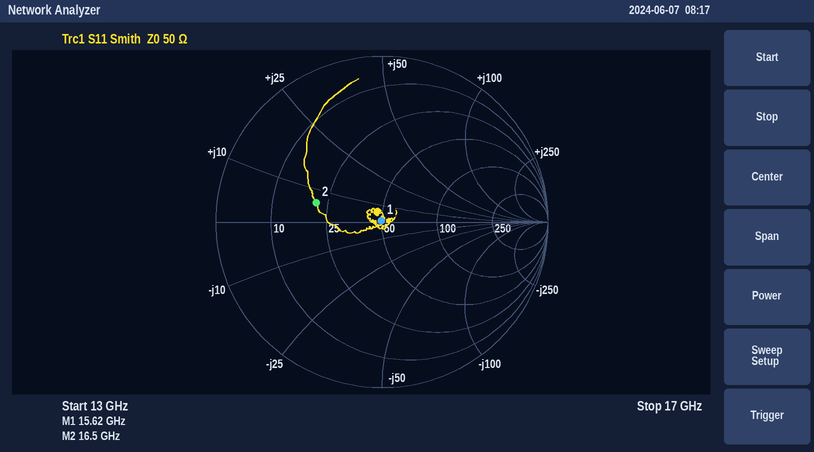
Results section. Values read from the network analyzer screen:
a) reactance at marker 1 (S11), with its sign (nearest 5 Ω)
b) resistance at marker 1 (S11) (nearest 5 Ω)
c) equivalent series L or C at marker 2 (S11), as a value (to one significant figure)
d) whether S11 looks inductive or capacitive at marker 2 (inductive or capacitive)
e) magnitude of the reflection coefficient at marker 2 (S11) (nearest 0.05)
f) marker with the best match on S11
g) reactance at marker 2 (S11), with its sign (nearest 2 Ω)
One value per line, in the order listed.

0 Ω
50 Ω
60 pH
inductive
0.40
marker 1
+6 Ω
